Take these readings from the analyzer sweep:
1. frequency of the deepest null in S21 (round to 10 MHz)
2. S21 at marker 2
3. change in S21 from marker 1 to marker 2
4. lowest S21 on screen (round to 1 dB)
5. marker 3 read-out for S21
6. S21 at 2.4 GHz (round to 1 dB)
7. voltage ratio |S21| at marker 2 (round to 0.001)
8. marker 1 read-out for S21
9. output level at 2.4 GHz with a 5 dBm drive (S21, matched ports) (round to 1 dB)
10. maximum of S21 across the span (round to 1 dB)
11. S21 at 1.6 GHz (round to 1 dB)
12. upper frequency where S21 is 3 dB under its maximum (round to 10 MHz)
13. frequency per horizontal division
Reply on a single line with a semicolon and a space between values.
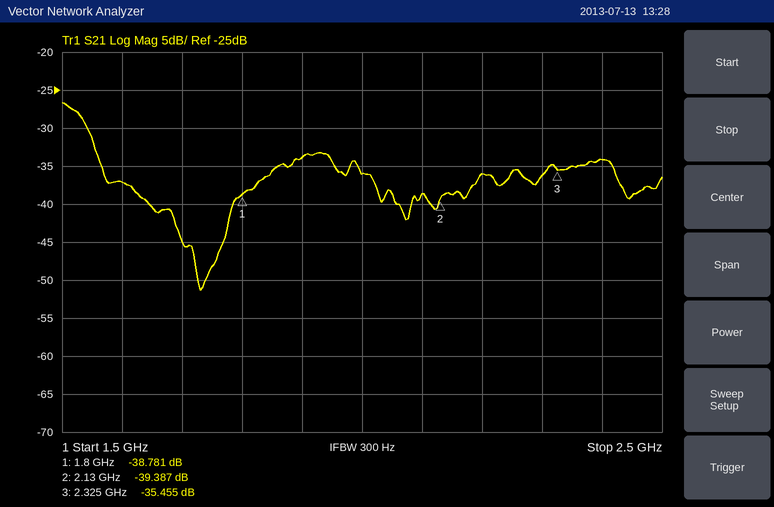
1.73 GHz; -39.387 dB; -0.606 dB; -51 dB; -35.455 dB; -34 dB; 0.011; -38.781 dB; -29 dBm; -27 dB; -37 dB; 1.54 GHz; 100 MHz
